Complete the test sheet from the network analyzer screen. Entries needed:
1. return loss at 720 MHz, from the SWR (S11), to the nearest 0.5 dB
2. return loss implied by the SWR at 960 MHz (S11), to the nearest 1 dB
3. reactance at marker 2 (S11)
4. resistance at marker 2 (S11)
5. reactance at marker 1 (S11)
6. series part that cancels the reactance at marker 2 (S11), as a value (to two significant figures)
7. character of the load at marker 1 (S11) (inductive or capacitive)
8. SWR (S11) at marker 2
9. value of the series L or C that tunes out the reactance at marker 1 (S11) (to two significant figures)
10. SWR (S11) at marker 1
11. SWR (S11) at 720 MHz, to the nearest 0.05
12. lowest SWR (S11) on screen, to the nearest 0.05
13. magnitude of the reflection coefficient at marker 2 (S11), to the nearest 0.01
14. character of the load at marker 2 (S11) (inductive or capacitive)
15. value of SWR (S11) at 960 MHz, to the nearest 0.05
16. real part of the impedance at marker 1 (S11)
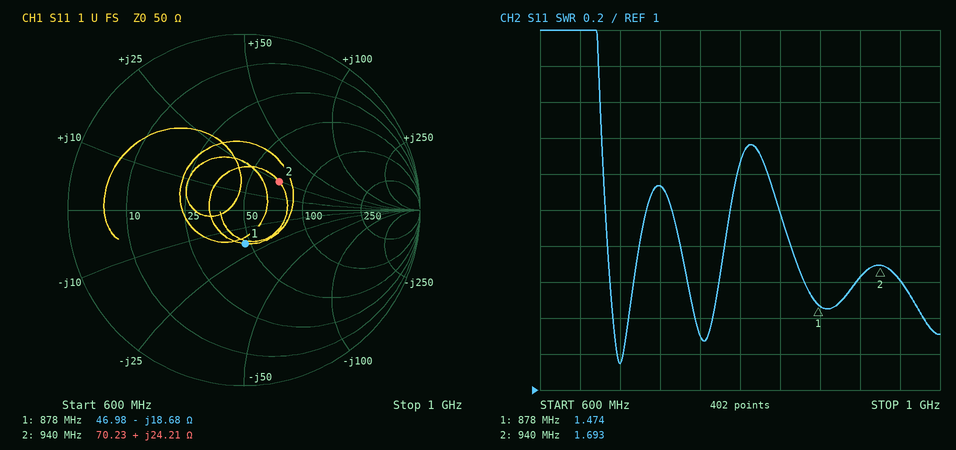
9.0 dB
13 dB
+24.21 Ω
70.23 Ω
-18.68 Ω
7.0 pF
capacitive
1.693
3.4 nH
1.474
2.15
1.15
0.26
inductive
1.60
46.98 Ω
